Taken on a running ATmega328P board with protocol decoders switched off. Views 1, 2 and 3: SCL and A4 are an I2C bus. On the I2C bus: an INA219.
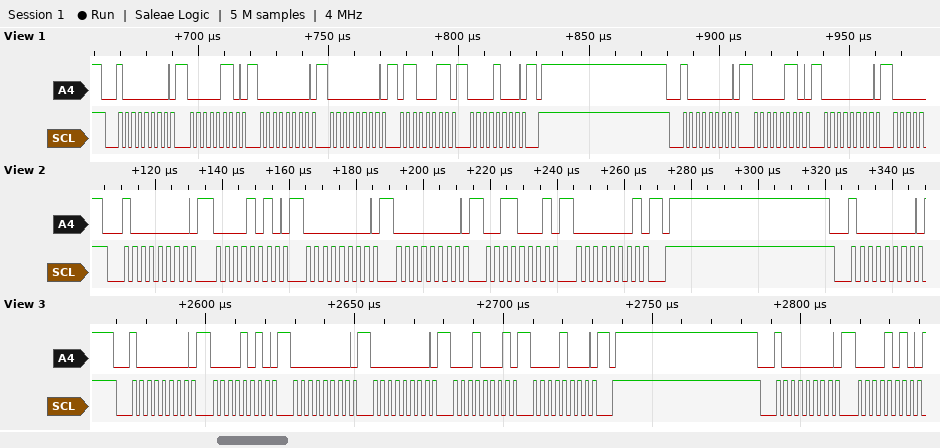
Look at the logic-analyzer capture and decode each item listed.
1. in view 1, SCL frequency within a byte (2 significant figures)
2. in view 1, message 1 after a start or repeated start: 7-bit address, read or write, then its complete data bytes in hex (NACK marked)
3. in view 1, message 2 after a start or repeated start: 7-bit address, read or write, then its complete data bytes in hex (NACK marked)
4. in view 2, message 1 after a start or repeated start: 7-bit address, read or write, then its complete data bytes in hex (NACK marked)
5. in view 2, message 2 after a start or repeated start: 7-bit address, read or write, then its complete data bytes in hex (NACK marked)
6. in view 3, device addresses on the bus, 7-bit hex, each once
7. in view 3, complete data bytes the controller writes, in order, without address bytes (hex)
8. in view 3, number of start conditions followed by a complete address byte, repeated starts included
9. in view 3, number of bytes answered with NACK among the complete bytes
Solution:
400 kHz
0x40 write: 06 00 00 63 08
0x40 write: 06 00
0x40 write: 0A 00 00 31 01
0x40 write
0x40
0A 00 00 11 08 0A
2
0
